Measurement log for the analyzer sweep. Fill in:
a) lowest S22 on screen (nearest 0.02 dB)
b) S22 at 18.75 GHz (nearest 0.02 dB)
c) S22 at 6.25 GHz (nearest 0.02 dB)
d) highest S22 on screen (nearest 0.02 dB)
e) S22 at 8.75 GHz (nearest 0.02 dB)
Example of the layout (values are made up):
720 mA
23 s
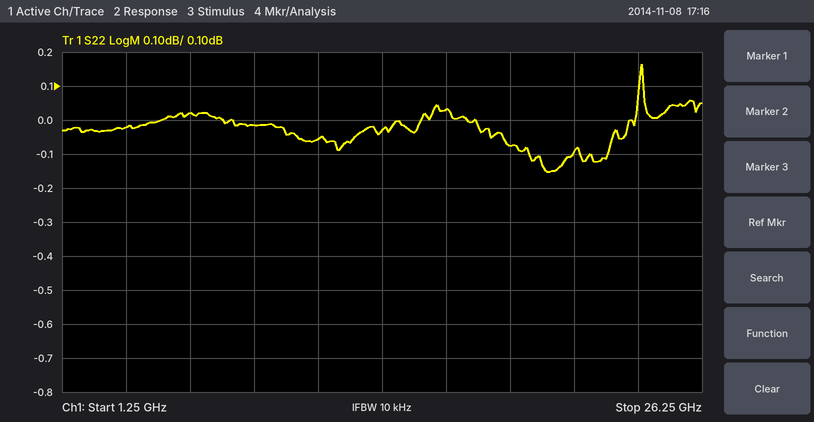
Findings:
-0.16 dB
-0.08 dB
0.02 dB
0.16 dB
-0.02 dB
